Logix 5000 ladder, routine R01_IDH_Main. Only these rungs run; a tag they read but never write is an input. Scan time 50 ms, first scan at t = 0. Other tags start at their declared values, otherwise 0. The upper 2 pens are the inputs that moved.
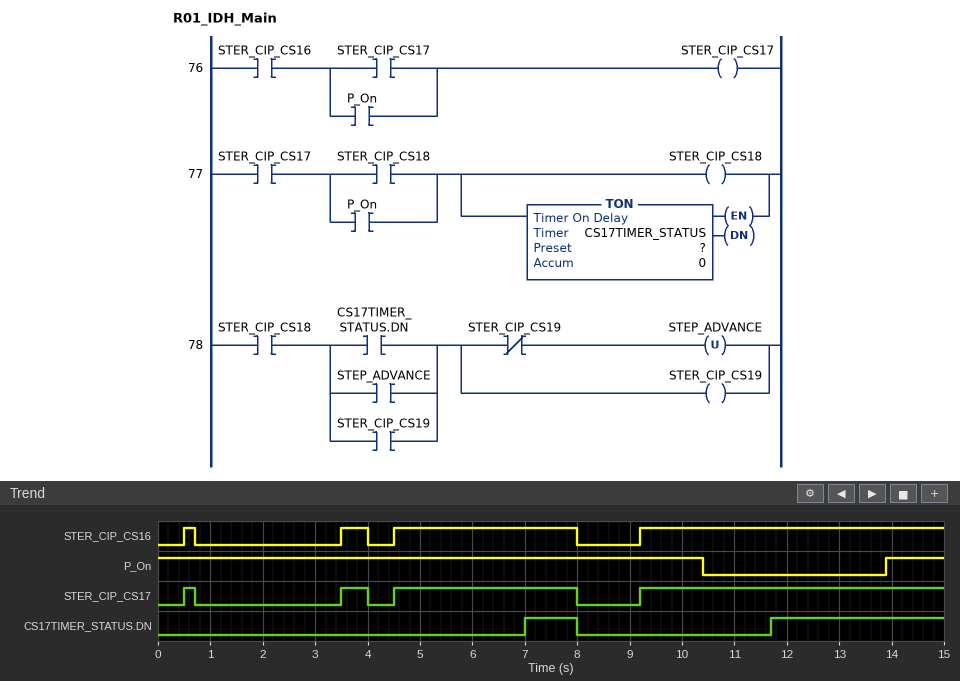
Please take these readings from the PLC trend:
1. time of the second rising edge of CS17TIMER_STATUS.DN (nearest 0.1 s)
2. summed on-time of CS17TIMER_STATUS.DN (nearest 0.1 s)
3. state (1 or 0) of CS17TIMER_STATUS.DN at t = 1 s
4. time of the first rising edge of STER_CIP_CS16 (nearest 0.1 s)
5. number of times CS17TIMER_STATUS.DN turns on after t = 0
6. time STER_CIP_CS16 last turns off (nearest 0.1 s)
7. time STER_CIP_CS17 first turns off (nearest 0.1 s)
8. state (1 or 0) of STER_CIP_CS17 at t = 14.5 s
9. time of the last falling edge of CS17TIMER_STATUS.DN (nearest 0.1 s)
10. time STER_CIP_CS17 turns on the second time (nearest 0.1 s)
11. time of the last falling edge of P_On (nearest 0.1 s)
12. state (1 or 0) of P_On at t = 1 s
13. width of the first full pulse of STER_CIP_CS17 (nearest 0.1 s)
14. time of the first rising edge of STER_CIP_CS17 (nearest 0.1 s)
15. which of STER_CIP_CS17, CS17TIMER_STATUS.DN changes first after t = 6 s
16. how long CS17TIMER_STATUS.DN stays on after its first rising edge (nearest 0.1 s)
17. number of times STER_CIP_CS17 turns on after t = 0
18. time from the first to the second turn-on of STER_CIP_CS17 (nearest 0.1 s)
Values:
11.7 s
4.3 s
0
0.5 s
2
8.0 s
0.7 s
1
8.0 s
3.5 s
10.4 s
1
0.2 s
0.5 s
CS17TIMER_STATUS.DN
1.0 s
4
3.0 s
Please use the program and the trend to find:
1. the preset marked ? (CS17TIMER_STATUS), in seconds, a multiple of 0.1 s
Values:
2.5 s
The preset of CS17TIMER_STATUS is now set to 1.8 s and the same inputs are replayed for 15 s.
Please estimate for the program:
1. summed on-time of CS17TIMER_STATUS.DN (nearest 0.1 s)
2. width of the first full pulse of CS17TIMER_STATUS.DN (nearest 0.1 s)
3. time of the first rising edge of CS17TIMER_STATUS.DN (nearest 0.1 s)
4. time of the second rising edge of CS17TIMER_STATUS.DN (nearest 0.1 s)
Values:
5.7 s
1.7 s
6.3 s
11.0 s
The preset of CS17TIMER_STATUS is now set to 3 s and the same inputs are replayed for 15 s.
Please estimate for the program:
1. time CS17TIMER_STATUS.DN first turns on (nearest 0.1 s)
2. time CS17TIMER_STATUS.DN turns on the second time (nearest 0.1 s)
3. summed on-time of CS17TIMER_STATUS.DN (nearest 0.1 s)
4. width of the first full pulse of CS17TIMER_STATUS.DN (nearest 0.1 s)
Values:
7.5 s
12.2 s
3.3 s
0.5 s
